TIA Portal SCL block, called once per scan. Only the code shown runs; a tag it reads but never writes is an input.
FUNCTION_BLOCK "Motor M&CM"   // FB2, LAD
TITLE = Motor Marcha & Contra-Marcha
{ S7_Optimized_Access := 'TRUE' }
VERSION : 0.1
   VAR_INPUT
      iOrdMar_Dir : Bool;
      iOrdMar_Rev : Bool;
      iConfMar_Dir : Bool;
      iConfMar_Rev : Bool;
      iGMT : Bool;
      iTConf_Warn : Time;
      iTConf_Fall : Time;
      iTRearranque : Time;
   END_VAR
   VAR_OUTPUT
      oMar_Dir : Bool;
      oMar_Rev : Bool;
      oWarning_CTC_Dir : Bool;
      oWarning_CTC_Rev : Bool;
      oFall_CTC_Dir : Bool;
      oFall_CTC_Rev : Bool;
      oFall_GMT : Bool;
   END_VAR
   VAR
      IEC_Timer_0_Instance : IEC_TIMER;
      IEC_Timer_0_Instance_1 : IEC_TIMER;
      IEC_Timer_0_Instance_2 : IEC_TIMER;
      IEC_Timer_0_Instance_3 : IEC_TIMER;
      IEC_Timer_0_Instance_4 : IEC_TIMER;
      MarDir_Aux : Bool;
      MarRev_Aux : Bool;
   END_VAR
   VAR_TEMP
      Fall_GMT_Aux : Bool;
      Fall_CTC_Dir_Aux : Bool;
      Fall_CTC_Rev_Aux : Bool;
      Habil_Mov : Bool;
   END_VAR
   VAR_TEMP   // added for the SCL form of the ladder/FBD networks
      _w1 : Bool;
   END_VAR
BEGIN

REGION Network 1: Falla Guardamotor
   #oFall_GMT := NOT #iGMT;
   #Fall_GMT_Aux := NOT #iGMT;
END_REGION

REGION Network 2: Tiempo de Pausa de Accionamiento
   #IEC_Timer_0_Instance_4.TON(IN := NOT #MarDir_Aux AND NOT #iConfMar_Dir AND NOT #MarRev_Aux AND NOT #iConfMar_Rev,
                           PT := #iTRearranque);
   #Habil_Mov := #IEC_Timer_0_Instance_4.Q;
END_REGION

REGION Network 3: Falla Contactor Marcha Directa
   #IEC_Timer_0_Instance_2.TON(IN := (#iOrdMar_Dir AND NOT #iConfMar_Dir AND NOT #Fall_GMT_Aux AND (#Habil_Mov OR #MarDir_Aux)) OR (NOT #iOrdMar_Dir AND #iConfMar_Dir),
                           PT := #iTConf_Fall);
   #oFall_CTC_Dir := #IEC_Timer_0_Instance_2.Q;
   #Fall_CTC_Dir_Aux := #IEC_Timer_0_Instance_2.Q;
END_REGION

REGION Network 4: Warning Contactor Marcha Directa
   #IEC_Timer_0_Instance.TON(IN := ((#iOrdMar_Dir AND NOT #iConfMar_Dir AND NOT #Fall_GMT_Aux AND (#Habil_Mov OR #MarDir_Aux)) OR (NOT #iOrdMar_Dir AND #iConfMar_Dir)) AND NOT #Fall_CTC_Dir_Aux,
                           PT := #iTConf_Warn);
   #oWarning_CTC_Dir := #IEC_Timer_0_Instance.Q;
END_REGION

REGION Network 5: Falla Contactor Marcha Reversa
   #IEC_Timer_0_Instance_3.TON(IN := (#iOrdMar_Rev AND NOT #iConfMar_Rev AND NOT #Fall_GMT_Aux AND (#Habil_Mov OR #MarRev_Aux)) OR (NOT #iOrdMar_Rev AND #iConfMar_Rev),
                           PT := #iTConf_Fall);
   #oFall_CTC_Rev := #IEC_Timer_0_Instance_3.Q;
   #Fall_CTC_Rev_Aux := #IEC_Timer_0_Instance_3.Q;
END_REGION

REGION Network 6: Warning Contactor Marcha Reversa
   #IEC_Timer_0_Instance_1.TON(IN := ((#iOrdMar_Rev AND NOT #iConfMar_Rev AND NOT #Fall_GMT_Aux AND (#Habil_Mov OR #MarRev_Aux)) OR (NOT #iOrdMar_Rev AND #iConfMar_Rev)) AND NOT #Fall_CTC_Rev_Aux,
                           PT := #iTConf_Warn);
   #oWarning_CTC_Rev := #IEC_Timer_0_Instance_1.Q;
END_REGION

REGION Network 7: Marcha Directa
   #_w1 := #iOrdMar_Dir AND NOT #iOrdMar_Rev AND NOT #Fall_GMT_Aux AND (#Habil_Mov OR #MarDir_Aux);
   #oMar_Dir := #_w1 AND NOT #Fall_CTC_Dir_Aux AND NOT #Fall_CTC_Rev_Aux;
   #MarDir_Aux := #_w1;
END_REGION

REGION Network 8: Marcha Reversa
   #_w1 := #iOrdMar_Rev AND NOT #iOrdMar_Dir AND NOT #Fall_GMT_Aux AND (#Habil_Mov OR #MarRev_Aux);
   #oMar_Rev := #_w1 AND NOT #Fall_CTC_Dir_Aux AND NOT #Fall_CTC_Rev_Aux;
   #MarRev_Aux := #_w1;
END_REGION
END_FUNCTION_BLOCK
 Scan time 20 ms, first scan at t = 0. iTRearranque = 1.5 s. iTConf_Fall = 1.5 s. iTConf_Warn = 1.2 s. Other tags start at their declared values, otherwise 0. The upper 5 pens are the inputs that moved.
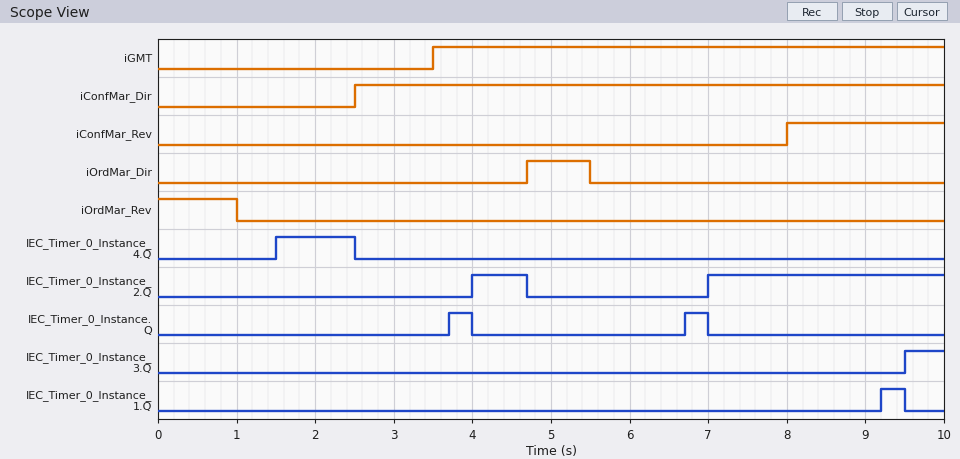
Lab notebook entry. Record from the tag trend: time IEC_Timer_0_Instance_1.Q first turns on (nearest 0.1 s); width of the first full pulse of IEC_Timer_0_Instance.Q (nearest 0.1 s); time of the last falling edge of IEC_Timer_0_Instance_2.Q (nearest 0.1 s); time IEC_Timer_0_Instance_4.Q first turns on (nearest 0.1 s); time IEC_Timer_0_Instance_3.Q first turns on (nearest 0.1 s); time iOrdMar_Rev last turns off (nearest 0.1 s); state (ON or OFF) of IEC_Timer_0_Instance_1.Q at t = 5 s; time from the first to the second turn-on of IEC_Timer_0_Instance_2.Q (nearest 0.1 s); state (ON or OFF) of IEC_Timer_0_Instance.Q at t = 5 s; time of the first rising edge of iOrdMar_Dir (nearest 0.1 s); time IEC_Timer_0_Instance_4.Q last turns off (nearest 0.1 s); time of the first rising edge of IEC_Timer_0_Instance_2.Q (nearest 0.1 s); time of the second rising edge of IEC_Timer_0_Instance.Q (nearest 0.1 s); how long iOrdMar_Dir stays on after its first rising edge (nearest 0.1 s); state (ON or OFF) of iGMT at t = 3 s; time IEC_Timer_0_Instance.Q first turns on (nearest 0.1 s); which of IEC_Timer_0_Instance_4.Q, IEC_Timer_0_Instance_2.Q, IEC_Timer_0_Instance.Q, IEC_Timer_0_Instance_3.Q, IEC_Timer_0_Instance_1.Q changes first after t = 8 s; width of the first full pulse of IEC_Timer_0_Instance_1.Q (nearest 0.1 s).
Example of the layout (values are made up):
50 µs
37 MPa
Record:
9.2 s
0.3 s
4.7 s
1.5 s
9.5 s
1.0 s
OFF
3.0 s
OFF
4.7 s
2.5 s
4.0 s
6.7 s
0.8 s
OFF
3.7 s
IEC_Timer_0_Instance_1.Q
0.3 s
